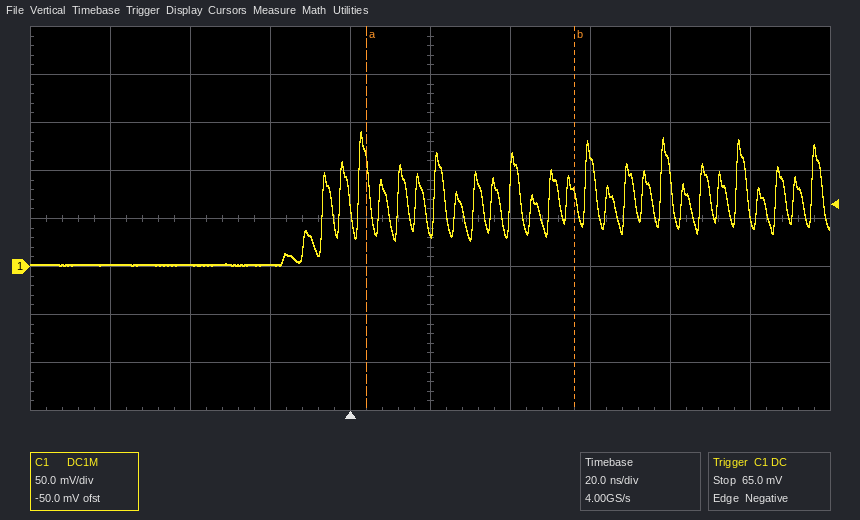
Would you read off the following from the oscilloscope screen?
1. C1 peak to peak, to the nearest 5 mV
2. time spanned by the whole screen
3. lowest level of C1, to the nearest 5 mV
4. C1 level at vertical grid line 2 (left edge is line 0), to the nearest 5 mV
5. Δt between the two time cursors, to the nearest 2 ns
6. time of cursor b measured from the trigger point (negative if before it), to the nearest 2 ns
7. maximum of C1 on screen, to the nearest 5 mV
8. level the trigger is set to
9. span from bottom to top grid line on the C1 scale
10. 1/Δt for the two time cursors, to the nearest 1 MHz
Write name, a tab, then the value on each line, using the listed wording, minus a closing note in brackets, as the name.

C1 peak to peak, to the nearest 5 mV	140 mV
time spanned by the whole screen	200 ns
lowest level of C1, to the nearest 5 mV	0 mV
C1 level at vertical grid line 2 (left edge is line 0), to the nearest 5 mV	0 mV
Δt between the two time cursors, to the nearest 2 ns	52 ns
time of cursor b measured from the trigger point (negative if before it), to the nearest 2 ns	+56 ns
maximum of C1 on screen, to the nearest 5 mV	140 mV
level the trigger is set to	65.0 mV
span from bottom to top grid line on the C1 scale	400 mV
1/Δt for the two time cursors, to the nearest 1 MHz	19 MHz
